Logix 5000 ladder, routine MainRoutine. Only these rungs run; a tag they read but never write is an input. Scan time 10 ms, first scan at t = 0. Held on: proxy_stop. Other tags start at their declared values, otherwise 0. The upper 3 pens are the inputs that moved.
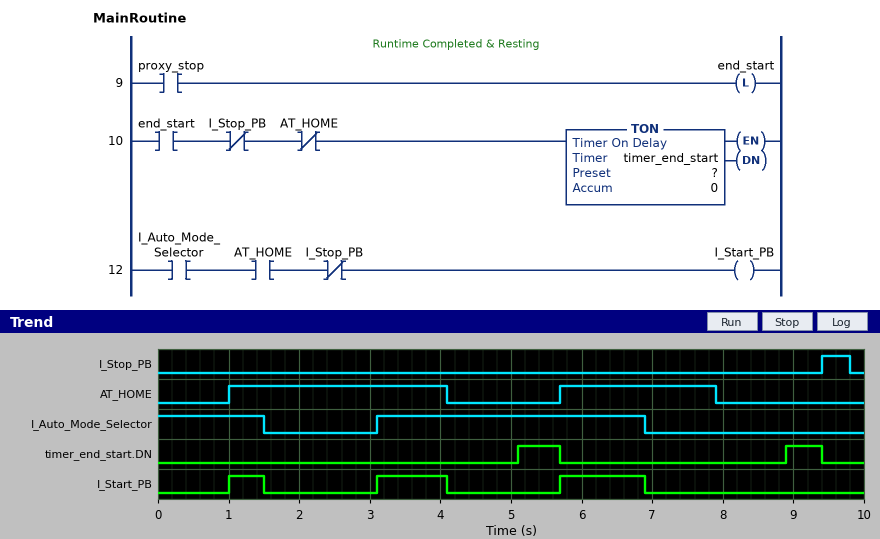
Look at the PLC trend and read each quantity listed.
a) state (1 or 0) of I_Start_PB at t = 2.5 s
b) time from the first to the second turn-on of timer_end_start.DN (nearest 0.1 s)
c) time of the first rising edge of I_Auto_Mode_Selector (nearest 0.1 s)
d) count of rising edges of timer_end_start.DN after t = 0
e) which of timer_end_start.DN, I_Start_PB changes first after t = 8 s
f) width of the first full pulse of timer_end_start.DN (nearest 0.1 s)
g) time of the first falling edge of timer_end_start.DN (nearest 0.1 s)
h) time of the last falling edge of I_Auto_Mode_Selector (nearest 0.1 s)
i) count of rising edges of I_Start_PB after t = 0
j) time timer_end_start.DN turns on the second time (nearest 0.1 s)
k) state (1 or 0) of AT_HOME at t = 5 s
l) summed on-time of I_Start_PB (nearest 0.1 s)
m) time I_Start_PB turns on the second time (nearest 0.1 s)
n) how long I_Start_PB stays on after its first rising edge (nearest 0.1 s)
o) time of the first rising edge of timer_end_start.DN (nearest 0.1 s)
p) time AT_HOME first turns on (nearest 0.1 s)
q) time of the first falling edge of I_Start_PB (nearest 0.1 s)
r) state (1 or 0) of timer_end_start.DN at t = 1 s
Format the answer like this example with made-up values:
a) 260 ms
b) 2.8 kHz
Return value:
a) 0
b) 3.8 s
c) 3.1 s
d) 2
e) timer_end_start.DN
f) 0.6 s
g) 5.7 s
h) 6.9 s
i) 3
j) 8.9 s
k) 0
l) 2.7 s
m) 3.1 s
n) 0.5 s
o) 5.1 s
p) 1.0 s
q) 1.5 s
r) 0
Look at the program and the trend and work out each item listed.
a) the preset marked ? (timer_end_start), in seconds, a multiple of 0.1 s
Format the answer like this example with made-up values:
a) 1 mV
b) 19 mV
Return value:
a) 1.0 s
